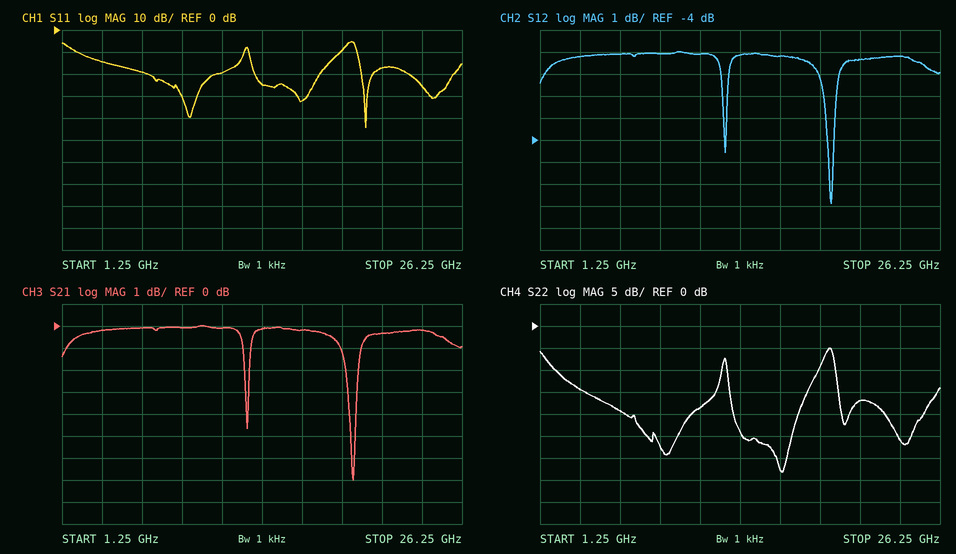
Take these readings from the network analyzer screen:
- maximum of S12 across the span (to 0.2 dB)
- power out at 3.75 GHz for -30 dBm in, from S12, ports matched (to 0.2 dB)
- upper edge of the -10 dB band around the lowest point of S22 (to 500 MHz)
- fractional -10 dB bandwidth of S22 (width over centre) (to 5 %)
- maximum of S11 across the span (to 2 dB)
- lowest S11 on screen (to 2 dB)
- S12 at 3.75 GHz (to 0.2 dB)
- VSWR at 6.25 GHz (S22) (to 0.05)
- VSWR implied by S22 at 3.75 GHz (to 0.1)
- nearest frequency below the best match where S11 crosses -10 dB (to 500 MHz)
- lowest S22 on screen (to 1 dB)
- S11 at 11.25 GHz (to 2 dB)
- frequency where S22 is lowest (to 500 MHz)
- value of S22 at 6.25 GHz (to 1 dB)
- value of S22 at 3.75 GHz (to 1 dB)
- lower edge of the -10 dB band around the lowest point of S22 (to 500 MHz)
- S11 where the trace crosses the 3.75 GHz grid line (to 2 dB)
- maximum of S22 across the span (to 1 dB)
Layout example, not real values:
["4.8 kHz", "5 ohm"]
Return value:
["0.0 dB", "-30.2 dBm", "18.5 GHz", "35 %", "-6 dB", "-44 dB", "-0.2 dB", "1.25", "1.5", "19.5 GHz", "-33 dB", "-20 dB", "16.5 GHz", "-19 dB", "-14 dB", "13.0 GHz", "-14 dB", "-5 dB"]
